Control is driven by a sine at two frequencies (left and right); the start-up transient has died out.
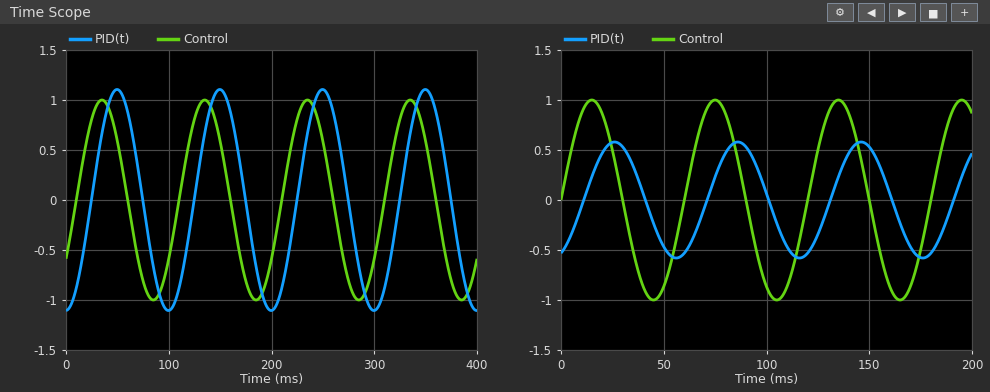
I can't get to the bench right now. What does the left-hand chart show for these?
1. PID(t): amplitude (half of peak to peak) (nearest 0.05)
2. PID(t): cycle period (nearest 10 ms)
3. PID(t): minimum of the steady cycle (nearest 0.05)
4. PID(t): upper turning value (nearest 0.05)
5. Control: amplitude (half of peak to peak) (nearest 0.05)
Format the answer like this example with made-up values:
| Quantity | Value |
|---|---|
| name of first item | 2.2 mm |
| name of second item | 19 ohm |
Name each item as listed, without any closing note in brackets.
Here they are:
| Quantity | Value |
|---|---|
| PID(t): amplitude (half of peak to peak) | 1.10 |
| PID(t): cycle period | 100 ms |
| PID(t): minimum of the steady cycle | -1.10 |
| PID(t): upper turning value | 1.10 |
| Control: amplitude (half of peak to peak) | 1.00 |
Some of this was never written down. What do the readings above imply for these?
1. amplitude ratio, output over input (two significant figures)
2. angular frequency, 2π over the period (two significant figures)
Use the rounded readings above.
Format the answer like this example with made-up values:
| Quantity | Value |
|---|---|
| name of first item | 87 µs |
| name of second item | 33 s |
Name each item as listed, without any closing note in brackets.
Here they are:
| Quantity | Value |
|---|---|
| amplitude ratio, output over input | 1.1 |
| angular frequency, 2π over the period | 0.063 rad/ms |
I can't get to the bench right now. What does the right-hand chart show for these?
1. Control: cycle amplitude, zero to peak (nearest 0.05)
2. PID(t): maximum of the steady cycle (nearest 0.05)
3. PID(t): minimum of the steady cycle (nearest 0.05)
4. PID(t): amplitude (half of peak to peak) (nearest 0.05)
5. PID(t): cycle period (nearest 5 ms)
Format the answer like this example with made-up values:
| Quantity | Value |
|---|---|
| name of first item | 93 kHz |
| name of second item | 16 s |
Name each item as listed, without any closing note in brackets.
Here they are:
| Quantity | Value |
|---|---|
| Control: cycle amplitude, zero to peak | 1.00 |
| PID(t): maximum of the steady cycle | 0.60 |
| PID(t): minimum of the steady cycle | -0.60 |
| PID(t): amplitude (half of peak to peak) | 0.60 |
| PID(t): cycle period | 60 ms |
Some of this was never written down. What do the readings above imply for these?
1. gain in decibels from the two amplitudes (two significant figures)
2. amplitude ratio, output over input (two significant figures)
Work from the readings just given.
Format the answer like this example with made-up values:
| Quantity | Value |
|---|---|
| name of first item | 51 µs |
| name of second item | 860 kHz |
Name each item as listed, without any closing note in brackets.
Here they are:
| Quantity | Value |
|---|---|
| gain in decibels from the two amplitudes | -4.4 dB |
| amplitude ratio, output over input | 0.60 |
